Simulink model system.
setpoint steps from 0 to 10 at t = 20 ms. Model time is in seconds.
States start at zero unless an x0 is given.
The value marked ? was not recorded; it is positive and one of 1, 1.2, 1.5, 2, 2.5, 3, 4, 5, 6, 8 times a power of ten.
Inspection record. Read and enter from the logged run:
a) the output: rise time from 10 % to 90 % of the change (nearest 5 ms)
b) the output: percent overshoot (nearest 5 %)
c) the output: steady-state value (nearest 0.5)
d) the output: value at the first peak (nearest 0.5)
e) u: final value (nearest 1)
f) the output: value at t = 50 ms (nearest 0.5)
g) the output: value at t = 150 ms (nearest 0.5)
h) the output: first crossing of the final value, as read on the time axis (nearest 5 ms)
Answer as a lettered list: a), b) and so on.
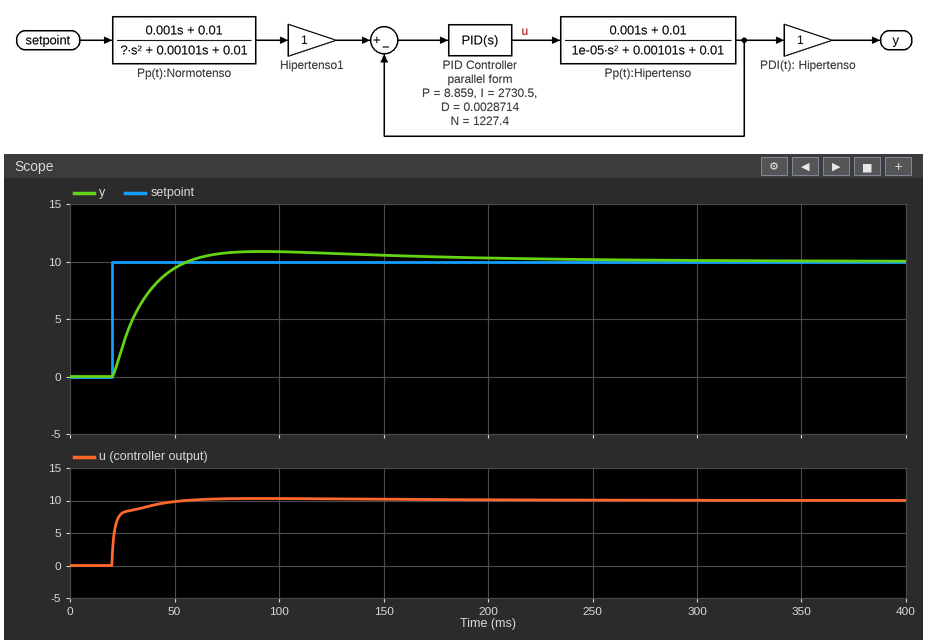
a) 25 ms
b) 10 %
c) 10.0
d) 11.0
e) 10
f) 9.5
g) 10.5
h) 55 ms
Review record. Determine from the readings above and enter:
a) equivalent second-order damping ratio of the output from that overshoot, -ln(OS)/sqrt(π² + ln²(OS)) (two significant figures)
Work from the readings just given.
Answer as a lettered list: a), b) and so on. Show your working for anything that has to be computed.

a) ln(0.1) = -2.303; 2.303 / sqrt(9.870 + 5.302) = 0.59
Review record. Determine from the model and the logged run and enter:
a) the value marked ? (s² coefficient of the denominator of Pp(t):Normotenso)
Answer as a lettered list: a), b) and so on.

a) 1.5e-05
